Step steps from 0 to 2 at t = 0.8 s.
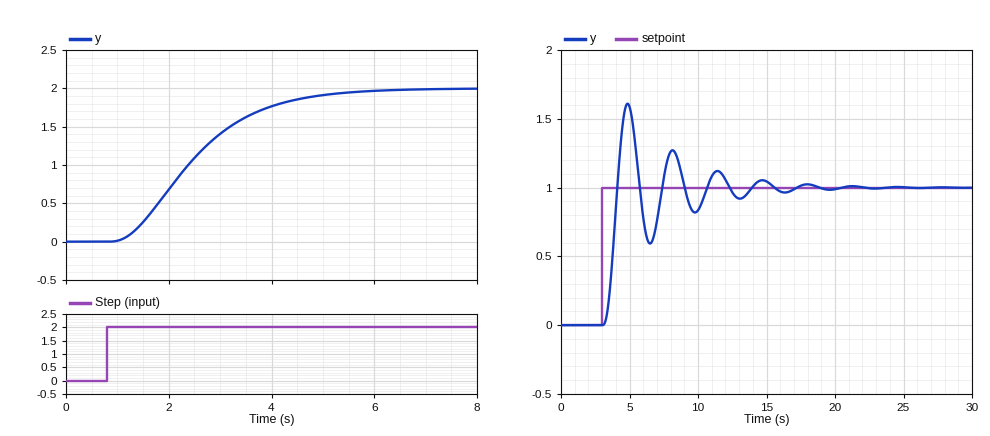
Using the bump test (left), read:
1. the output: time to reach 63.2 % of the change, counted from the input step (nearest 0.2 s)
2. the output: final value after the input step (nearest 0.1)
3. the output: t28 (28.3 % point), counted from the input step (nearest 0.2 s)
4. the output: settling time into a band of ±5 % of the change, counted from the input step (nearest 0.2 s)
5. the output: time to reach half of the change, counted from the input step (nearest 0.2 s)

2.0 s
2.0
1.0 s
4.0 s
1.6 s
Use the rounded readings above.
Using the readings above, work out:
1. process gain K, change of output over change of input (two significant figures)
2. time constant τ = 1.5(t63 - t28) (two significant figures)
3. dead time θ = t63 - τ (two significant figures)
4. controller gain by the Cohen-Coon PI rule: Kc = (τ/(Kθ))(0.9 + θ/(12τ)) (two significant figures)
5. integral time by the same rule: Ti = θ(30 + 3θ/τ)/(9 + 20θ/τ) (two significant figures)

1.0
1.5 s
0.50 s
2.8
0.99 s
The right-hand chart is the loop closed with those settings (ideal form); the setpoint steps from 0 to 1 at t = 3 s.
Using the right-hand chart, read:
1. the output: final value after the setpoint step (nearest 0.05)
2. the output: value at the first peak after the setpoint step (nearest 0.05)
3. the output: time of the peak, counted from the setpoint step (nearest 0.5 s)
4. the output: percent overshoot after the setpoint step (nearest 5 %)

1.00
1.60
2.0 s
60 %
